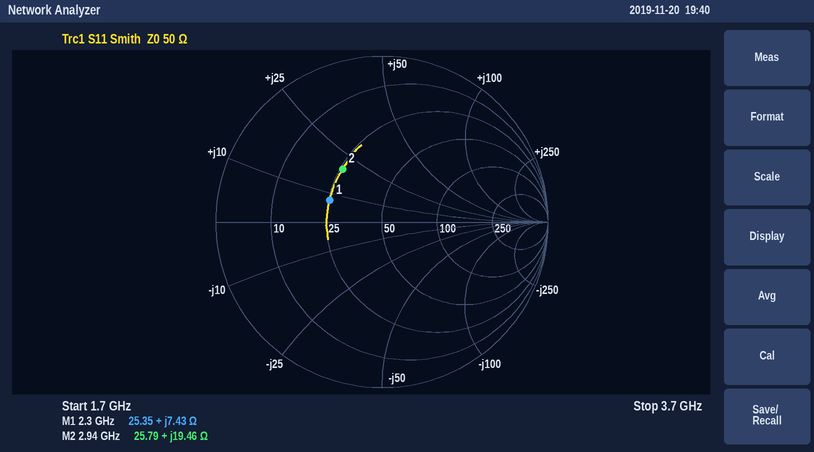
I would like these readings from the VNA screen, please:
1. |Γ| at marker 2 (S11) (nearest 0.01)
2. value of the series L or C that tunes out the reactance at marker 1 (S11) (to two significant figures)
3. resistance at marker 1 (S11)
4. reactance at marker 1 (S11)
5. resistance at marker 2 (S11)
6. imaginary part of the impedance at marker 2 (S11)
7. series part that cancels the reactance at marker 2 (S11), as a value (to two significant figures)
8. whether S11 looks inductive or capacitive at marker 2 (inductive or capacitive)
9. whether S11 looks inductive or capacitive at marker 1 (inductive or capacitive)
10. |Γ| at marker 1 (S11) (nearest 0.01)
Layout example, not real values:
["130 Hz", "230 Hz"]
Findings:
["0.40", "9.3 pF", "25.35 Ω", "+7.43 Ω", "25.79 Ω", "+19.46 Ω", "2.8 pF", "inductive", "inductive", "0.34"]
